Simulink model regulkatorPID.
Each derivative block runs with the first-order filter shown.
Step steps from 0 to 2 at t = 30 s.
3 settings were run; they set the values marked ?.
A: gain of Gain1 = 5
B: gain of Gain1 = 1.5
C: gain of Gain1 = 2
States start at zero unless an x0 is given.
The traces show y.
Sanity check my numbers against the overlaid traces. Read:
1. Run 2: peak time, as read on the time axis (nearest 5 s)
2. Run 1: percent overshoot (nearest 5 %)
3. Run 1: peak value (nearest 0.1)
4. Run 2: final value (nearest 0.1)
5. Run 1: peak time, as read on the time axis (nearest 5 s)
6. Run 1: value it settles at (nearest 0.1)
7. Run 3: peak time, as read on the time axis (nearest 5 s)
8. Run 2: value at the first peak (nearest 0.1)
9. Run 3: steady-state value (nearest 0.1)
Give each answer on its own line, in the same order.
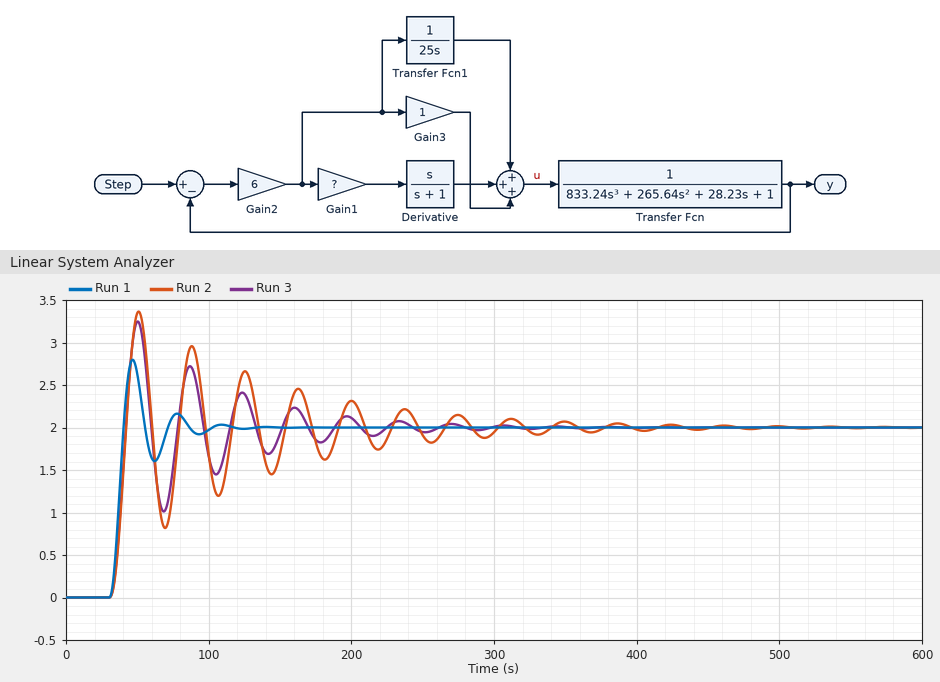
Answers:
50 s
40 %
2.8
2.0
45 s
2.0
50 s
3.4
2.0
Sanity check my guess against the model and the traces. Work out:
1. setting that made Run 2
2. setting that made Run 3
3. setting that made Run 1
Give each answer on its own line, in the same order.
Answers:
B
C
A
